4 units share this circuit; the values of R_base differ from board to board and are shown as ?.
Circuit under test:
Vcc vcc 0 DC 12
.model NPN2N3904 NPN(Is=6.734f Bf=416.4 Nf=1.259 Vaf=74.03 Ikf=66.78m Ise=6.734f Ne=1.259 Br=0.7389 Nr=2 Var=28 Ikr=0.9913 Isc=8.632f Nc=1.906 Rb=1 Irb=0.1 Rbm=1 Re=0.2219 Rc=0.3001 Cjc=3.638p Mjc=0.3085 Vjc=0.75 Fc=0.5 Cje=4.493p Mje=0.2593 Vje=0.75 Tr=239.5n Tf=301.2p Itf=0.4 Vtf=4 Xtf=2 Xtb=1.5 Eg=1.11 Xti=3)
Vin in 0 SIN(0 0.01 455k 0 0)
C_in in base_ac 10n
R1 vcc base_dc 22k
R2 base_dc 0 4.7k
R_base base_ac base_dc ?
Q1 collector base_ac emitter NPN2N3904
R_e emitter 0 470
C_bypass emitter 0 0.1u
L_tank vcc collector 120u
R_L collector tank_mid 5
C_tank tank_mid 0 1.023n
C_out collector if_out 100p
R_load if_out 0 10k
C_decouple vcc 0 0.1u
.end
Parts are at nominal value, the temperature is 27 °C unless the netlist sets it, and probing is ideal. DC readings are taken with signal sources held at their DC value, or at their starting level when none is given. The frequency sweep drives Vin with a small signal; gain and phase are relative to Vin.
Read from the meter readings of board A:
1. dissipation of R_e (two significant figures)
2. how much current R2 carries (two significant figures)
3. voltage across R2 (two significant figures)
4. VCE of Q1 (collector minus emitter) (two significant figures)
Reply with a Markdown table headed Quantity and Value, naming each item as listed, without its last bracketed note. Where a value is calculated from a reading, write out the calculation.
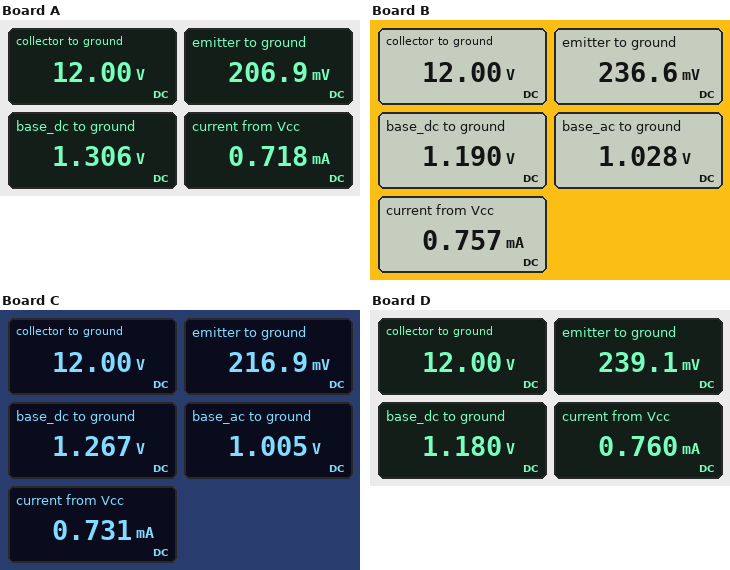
| Quantity | Value |
|---|---|
| dissipation of R_e | (206.9 mV)^2 / 470 Ω = 91 µW |
| how much current R2 carries | (1.306 V) / 4.7 kΩ = 280 µA |
| voltage across R2 | 1.306 V = 1.3 V |
| VCE of Q1 (collector minus emitter) | 12 V - 206.9 mV = 12 V |
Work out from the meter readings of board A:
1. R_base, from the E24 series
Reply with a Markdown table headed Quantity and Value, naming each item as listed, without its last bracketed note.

| Quantity | Value |
|---|---|
| R_base, from the E24 series | 1.5 kΩ |
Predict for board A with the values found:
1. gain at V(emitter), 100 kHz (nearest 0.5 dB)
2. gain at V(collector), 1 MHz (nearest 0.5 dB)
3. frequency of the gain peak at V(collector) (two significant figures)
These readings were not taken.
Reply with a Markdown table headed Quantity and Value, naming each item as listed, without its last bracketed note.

| Quantity | Value |
|---|---|
| gain at V(emitter), 100 kHz | -17.5 dB |
| gain at V(collector), 1 MHz | 2.5 dB |
| frequency of the gain peak at V(collector) | 450 kHz |
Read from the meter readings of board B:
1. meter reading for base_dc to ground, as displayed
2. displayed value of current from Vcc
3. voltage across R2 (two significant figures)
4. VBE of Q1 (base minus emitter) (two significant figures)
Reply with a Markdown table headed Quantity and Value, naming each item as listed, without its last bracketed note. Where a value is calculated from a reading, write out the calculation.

| Quantity | Value |
|---|---|
| meter reading for base_dc to ground, as displayed | 1.190 V |
| displayed value of current from Vcc | 0.757 mA |
| voltage across R2 | 1.19 V = 1.2 V |
| VBE of Q1 (base minus emitter) | 1.028 V - 236.6 mV = 790 mV |
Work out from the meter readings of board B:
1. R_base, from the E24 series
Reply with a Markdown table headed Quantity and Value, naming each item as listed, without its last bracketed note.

| Quantity | Value |
|---|---|
| R_base, from the E24 series | 680 Ω |
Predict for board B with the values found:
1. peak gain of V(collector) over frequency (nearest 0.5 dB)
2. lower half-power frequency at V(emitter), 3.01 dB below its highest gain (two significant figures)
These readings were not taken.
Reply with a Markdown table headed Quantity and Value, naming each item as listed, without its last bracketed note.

| Quantity | Value |
|---|---|
| peak gain of V(collector) over frequency | 35.0 dB |
| lower half-power frequency at V(emitter), 3.01 dB below its highest gain | 3.3 kHz |
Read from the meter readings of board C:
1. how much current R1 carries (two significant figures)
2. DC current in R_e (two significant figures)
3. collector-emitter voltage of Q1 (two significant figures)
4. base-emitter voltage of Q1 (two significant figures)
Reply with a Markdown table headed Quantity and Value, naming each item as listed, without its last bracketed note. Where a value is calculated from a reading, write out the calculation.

| Quantity | Value |
|---|---|
| how much current R1 carries | (12 V - 1.267 V) / 22 kΩ = 490 µA |
| DC current in R_e | (216.9 mV) / 470 Ω = 460 µA |
| collector-emitter voltage of Q1 | 12 V - 216.9 mV = 12 V |
| base-emitter voltage of Q1 | 1.005 V - 216.9 mV = 790 mV |
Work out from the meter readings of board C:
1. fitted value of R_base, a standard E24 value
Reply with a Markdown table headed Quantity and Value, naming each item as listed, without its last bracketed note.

| Quantity | Value |
|---|---|
| fitted value of R_base, a standard E24 value | 1.2 kΩ |
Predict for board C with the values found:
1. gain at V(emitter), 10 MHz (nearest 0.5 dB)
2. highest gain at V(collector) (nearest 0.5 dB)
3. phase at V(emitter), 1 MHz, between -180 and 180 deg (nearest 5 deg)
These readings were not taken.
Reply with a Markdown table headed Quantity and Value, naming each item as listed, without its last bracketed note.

| Quantity | Value |
|---|---|
| gain at V(emitter), 10 MHz | -53.0 dB |
| highest gain at V(collector) | 34.5 dB |
| phase at V(emitter), 1 MHz, between -180 and 180 deg | -80 deg |
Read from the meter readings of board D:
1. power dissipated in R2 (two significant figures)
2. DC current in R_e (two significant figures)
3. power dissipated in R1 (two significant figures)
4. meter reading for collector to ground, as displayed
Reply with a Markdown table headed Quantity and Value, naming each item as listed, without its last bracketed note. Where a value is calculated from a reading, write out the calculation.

| Quantity | Value |
|---|---|
| power dissipated in R2 | (1.18 V)^2 / 4.7 kΩ = 300 µW |
| DC current in R_e | (239.1 mV) / 470 Ω = 510 µA |
| power dissipated in R1 | (12 V - 1.18 V)^2 / 22 kΩ = 5.3 mW |
| meter reading for collector to ground, as displayed | 12.00 V |
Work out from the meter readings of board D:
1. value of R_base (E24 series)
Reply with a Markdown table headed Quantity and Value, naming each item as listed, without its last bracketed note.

| Quantity | Value |
|---|---|
| value of R_base | 620 Ω |
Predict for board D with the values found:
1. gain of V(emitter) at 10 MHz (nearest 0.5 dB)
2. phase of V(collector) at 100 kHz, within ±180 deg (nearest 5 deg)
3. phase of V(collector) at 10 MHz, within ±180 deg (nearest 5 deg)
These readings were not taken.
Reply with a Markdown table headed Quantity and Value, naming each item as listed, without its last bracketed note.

| Quantity | Value |
|---|---|
| gain of V(emitter) at 10 MHz | -52.0 dB |
| phase of V(collector) at 100 kHz, within ±180 deg | -35 deg |
| phase of V(collector) at 10 MHz, within ±180 deg | 110 deg |
